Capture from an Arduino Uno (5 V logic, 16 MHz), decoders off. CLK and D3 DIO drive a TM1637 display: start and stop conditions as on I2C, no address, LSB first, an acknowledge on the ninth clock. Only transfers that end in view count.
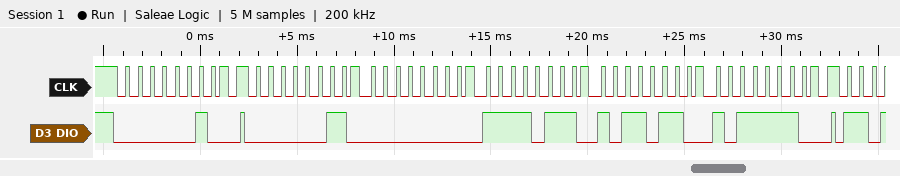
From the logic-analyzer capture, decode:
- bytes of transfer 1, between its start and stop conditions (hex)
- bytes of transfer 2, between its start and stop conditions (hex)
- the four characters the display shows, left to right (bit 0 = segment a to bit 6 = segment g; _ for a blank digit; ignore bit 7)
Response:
40
C0 00 EF 6D 7D
_956
